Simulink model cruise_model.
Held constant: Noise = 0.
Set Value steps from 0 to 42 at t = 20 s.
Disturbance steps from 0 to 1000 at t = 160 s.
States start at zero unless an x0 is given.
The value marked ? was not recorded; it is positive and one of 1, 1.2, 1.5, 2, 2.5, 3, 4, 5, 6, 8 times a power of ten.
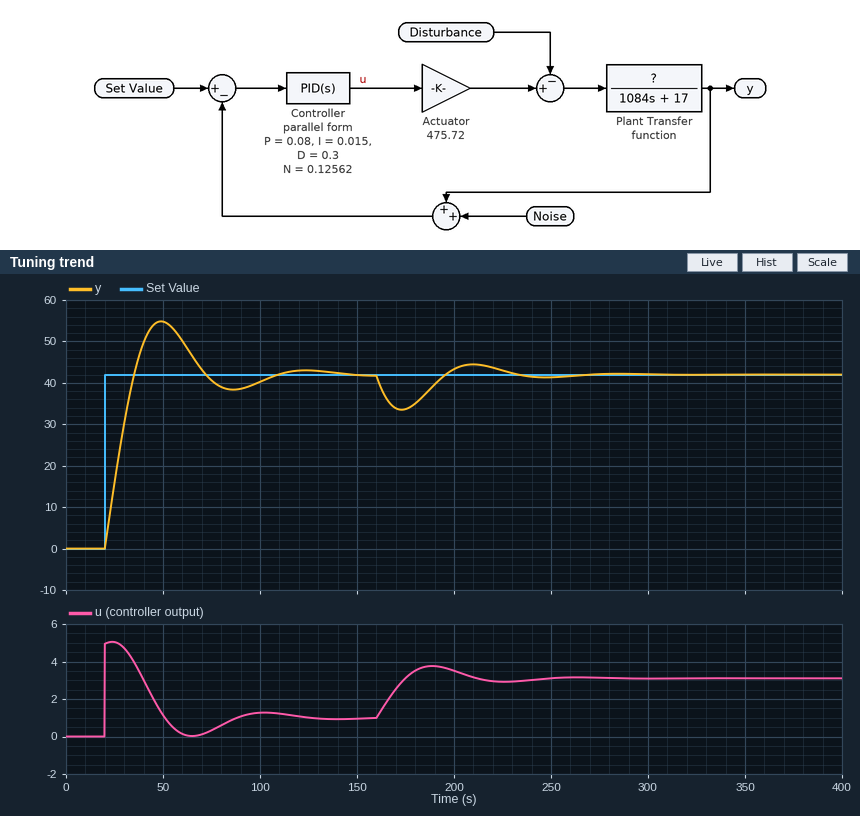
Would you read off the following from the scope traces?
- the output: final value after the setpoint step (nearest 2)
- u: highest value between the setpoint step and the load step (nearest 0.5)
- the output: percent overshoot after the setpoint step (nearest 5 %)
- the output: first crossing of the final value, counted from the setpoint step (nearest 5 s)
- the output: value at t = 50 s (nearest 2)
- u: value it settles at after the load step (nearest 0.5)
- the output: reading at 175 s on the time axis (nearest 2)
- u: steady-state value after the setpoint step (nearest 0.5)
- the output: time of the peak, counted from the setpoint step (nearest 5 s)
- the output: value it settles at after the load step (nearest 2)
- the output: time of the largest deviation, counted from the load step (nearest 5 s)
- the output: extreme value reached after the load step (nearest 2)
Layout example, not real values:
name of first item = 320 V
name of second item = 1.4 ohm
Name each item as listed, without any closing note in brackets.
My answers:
the output: final value after the setpoint step = 42
u: highest value between the setpoint step and the load step = 5.0
the output: percent overshoot after the setpoint step = 30 %
the output: first crossing of the final value, counted from the setpoint step = 15 s
the output: value at t = 50 s = 54
u: value it settles at after the load step = 3.0
the output: reading at 175 s on the time axis = 34
u: steady-state value after the setpoint step = 1.0
the output: time of the peak, counted from the setpoint step = 30 s
the output: value it settles at after the load step = 42
the output: time of the largest deviation, counted from the load step = 15 s
the output: extreme value reached after the load step = 34
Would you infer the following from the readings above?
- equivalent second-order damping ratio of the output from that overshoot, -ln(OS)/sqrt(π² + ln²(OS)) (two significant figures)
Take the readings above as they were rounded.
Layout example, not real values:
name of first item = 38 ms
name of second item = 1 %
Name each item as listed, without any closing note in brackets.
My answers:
equivalent second-order damping ratio of the output from that overshoot, -ln(OS)/sqrt(π² + ln²(OS)) = 0.36
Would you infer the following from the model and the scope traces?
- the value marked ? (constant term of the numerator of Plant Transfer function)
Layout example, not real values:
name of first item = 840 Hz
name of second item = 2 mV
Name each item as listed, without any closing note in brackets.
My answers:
the value marked ? = 1.5
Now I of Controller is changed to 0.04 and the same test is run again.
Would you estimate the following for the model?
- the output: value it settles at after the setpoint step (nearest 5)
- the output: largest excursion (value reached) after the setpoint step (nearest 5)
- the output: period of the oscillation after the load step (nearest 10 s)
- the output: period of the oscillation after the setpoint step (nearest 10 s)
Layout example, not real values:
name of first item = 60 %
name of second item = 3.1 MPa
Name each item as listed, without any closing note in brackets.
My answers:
the output: value it settles at after the setpoint step = 40
the output: largest excursion (value reached) after the setpoint step = 60
the output: period of the oscillation after the load step = 40 s
the output: period of the oscillation after the setpoint step = 40 s
